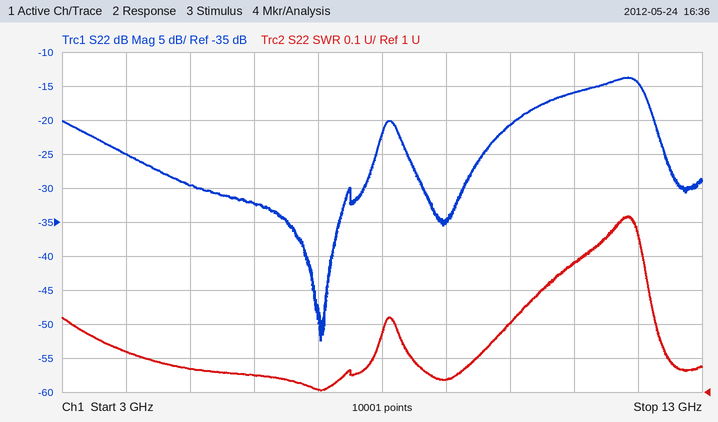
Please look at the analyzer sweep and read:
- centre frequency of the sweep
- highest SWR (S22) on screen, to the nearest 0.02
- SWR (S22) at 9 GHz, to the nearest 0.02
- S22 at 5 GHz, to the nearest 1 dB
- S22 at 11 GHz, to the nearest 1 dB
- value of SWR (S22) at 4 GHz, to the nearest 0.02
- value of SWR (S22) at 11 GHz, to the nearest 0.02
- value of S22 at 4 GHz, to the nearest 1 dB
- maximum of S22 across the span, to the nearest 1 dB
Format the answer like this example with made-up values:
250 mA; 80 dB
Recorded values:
8 GHz; 1.52; 1.04; -30 dB; -16 dB; 1.12; 1.38; -25 dB; -14 dB
